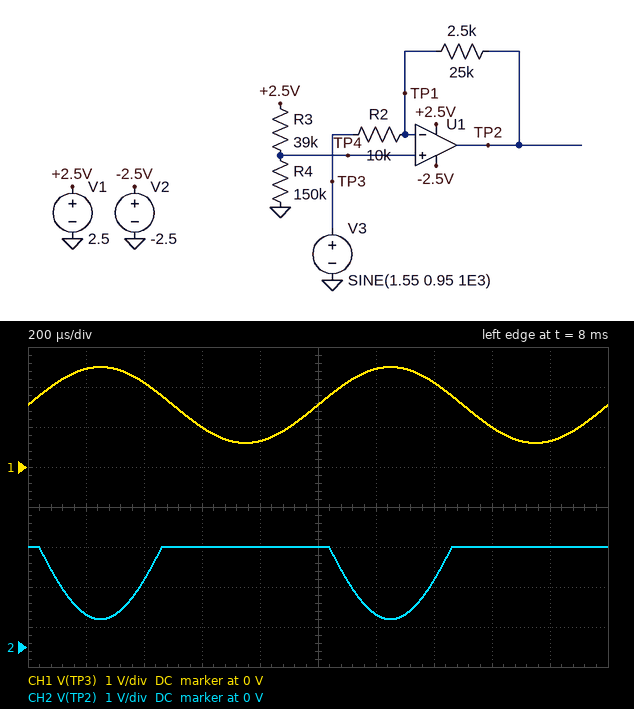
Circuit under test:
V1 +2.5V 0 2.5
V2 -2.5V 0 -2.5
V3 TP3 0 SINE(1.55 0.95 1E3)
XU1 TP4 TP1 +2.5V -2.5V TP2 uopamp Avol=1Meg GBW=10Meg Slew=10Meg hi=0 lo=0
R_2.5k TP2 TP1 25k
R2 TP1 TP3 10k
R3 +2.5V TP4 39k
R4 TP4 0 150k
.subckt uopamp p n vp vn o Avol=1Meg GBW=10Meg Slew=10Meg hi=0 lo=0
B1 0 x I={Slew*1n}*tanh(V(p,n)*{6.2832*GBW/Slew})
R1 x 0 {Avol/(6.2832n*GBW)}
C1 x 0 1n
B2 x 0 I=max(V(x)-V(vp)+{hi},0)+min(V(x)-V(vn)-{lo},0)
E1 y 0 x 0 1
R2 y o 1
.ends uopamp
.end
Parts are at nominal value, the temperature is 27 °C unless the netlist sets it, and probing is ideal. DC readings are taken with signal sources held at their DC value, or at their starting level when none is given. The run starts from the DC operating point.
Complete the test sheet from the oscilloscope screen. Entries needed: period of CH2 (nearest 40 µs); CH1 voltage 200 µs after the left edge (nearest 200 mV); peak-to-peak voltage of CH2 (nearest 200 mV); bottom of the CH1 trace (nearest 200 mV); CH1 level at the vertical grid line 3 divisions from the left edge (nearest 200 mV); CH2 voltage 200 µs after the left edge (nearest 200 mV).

1.00 ms
2.4 V
1.8 V
600 mV
1.0 V
800 mV
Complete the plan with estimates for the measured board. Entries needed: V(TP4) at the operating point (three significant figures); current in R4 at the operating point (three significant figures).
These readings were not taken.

1.98 V
13.2 µA
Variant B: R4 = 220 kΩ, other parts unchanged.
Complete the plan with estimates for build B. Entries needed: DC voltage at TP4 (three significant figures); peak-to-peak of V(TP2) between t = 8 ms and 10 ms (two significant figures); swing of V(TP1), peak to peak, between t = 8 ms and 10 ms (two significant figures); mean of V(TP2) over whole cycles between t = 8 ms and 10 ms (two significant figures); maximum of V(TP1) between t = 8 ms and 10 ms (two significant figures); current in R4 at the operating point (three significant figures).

2.12 V
1.3 V
980 mV
2.2 V
2.1 V
9.65 µA
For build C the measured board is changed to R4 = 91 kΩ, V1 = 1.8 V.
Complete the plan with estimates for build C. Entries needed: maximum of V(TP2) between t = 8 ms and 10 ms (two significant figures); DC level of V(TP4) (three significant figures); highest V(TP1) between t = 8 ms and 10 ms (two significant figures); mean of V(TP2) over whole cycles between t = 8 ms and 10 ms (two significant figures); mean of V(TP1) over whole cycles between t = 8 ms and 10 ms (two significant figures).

1.8 V
1.26 V
1.3 V
300 mV
1.2 V
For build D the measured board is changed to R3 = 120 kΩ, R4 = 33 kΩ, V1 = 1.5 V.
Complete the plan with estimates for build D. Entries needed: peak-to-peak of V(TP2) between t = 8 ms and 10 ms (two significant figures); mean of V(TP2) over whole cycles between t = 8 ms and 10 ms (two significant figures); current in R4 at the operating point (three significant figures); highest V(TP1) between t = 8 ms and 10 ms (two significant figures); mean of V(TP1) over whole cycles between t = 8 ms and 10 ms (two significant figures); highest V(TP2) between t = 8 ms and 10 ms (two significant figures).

2.1 V
-1.9 V
9.80 µA
1.1 V
570 mV
-370 mV
